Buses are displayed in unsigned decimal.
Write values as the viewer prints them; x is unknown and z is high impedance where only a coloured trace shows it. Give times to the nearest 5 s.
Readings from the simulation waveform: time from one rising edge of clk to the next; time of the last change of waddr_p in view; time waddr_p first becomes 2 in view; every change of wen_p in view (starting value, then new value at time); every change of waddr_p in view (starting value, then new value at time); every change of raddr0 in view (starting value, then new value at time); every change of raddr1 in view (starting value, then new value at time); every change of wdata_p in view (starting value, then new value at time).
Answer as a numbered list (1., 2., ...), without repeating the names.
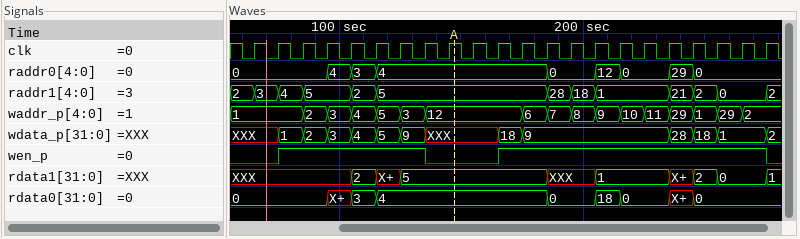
1. 10 s
2. 265 s
3. 85 s
4. 0, 1 at 75 s, 0 at 135 s, 1 at 165 s, 0 at 275 s
5. 1, 2 at 85 s, 3 at 95 s, 4 at 105 s, 5 at 115 s, 3 at 125 s, 12 at 135 s, 6 at 175 s, 7 at 185 s, 8 at 195 s, 9 at 205 s, 10 at 215 s, 11 at 225 s, 29 at 235 s, 1 at 245 s, 29 at 255 s, 2 at 265 s
6. 0, 4 at 95 s, 3 at 105 s, 4 at 115 s, 0 at 185 s, 12 at 205 s, 0 at 215 s, 29 at 235 s, 0 at 245 s
7. 2, 3 at 65 s, 4 at 75 s, 5 at 85 s, 2 at 105 s, 5 at 115 s, 28 at 185 s, 18 at 195 s, 1 at 205 s, 21 at 235 s, 2 at 245 s, 0 at 255 s, 2 at 275 s
8. XXX, 1 at 75 s, 2 at 85 s, 3 at 95 s, 4 at 105 s, 5 at 115 s, 9 at 125 s, XXX at 135 s, 18 at 165 s, 9 at 175 s, 28 at 235 s, 18 at 245 s, 1 at 255 s, 2 at 275 s
